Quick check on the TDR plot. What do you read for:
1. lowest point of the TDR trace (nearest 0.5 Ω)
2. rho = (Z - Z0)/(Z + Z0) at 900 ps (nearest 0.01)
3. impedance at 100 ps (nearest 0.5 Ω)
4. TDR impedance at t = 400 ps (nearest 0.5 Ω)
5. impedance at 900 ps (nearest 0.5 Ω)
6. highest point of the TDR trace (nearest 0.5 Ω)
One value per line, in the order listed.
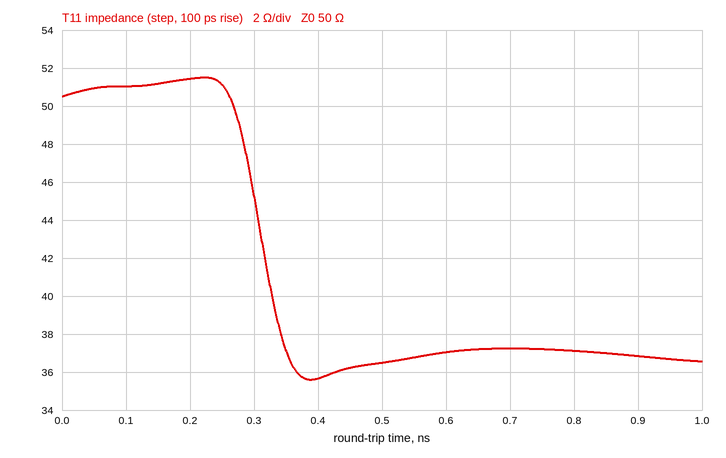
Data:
35.5 Ω
-0.15
51.0 Ω
35.5 Ω
37.0 Ω
51.5 Ω
